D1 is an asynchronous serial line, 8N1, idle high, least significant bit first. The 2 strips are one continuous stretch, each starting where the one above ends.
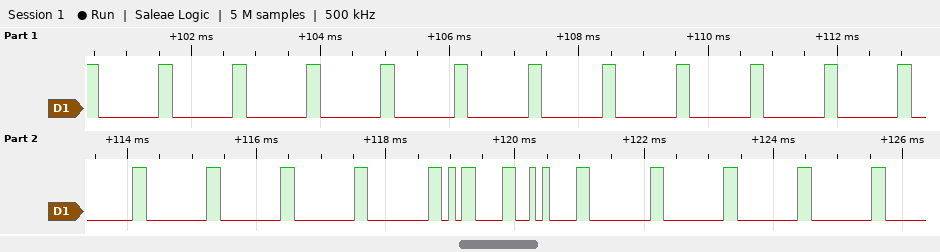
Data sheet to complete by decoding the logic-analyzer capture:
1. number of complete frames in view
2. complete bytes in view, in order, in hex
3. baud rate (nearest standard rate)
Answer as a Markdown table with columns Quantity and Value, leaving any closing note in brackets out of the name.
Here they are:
| Quantity | Value |
|---|---|
| number of complete frames in view | 22 |
| complete bytes in view, in order, in hex | 00 00 00 00 00 00 00 00 00 00 00 00 00 00 00 00 0D 0A 00 00 00 00 |
| baud rate | 9600 baud |
